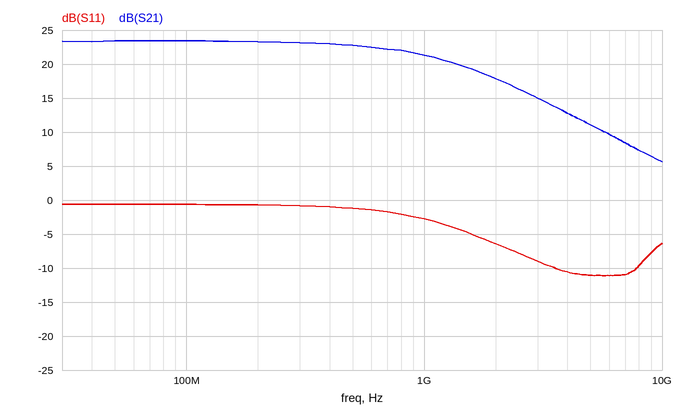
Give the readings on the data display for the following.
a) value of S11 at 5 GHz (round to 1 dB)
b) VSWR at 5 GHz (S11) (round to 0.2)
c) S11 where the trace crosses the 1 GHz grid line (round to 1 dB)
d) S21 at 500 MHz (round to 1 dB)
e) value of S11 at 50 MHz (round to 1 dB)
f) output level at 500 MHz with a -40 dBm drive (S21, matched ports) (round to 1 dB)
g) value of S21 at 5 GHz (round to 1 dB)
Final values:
-11 dB
1.8
-3 dB
23 dB
-1 dB
-17 dBm
11 dB
